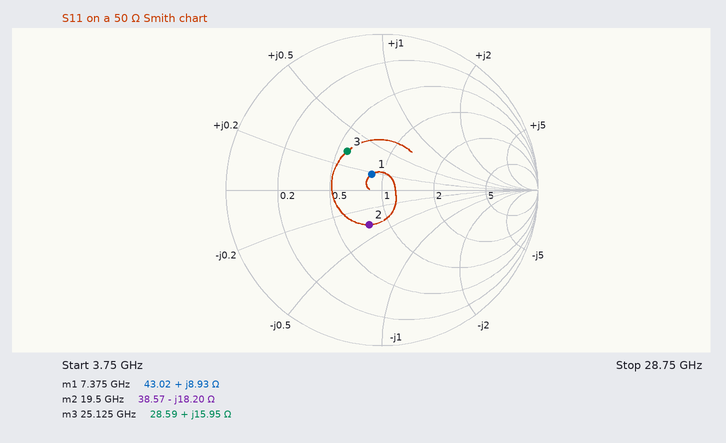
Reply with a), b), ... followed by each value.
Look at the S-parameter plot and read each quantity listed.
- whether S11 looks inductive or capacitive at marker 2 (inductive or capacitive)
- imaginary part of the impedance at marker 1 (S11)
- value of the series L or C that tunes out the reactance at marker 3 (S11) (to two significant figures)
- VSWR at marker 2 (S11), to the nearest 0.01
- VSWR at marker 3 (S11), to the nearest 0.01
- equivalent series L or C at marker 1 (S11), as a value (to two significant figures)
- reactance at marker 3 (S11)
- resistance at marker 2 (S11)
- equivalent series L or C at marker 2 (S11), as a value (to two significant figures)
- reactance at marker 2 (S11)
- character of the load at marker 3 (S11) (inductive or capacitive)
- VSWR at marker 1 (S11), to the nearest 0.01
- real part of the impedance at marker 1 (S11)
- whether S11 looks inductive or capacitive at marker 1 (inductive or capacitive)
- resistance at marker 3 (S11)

a) capacitive
b) +8.93 Ω
c) 400 fF
d) 1.62
e) 2.00
f) 190 pH
g) +15.95 Ω
h) 38.57 Ω
i) 450 fF
j) -18.20 Ω
k) inductive
l) 1.28
m) 43.02 Ω
n) inductive
o) 28.59 Ω
